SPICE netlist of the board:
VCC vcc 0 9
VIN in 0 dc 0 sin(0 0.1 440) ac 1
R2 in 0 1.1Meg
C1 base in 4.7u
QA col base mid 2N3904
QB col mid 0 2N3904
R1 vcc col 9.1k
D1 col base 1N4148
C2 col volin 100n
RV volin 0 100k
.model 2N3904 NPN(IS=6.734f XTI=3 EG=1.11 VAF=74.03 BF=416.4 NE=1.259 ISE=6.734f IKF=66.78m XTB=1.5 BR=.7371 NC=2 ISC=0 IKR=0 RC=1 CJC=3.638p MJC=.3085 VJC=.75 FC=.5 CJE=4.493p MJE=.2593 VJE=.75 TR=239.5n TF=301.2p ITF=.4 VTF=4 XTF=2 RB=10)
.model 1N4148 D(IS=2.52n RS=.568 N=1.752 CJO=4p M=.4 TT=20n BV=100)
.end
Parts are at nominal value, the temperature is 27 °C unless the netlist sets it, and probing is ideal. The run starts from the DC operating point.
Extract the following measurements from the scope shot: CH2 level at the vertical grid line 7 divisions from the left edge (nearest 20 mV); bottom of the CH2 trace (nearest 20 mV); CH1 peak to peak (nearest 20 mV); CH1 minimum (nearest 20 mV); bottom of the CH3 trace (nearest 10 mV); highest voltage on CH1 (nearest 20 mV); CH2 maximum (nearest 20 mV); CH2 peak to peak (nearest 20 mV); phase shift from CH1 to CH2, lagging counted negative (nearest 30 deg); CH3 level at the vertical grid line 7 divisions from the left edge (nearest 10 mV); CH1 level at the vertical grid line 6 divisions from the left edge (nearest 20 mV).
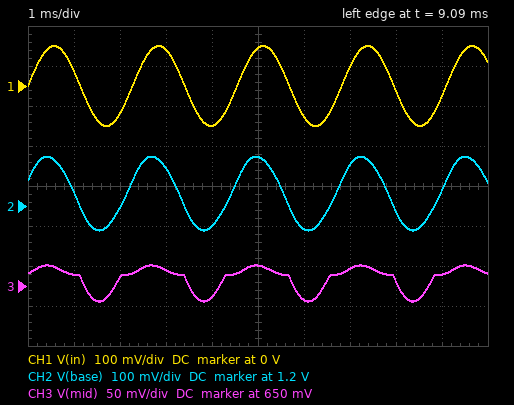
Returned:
1.30 V
1.14 V
200 mV
-100 mV
630 mV
100 mV
1.32 V
180 mV
30 deg
670 mV
-80 mV
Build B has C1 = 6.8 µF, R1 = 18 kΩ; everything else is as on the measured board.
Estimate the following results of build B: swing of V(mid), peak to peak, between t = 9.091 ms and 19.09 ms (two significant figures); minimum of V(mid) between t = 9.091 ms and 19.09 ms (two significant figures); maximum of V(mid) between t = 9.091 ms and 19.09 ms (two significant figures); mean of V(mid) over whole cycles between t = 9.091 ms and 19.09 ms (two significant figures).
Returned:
53 mV
610 mV
660 mV
640 mV
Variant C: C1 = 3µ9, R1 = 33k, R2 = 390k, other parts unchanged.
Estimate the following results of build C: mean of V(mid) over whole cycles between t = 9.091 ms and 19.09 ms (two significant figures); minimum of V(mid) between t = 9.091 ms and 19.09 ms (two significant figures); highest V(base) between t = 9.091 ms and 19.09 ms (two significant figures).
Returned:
620 mV
590 mV
1.3 V
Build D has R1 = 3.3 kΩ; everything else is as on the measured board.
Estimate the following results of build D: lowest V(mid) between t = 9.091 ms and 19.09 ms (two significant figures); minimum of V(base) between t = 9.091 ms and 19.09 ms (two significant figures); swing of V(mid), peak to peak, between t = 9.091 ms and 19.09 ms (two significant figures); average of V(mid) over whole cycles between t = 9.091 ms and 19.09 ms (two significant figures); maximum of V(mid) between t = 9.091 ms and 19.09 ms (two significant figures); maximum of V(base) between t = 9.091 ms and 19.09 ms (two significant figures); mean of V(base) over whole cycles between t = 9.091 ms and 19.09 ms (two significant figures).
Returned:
670 mV
1.2 V
29 mV
690 mV
700 mV
1.4 V
1.3 V
